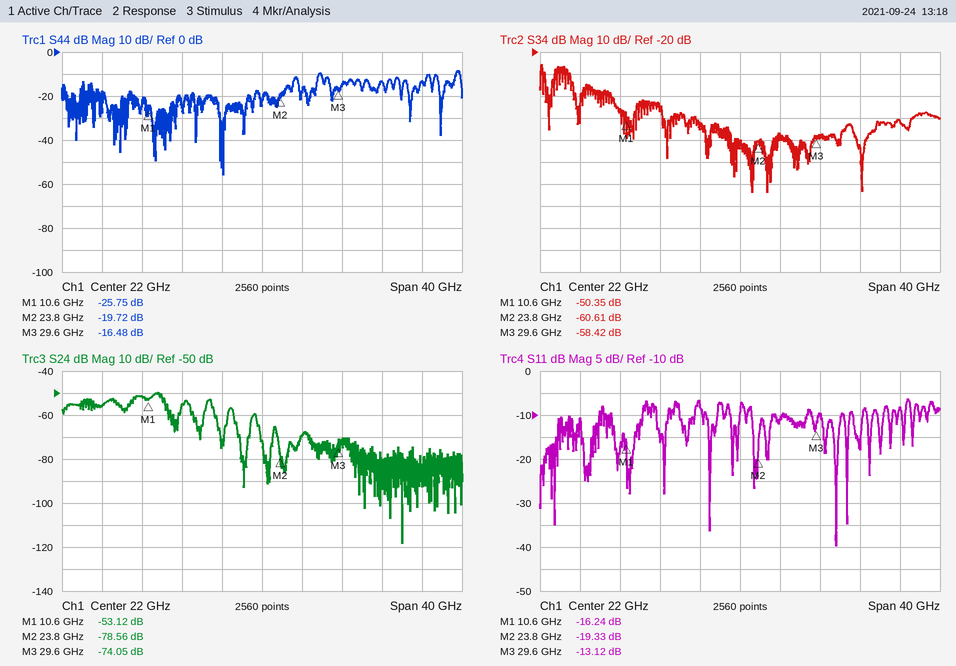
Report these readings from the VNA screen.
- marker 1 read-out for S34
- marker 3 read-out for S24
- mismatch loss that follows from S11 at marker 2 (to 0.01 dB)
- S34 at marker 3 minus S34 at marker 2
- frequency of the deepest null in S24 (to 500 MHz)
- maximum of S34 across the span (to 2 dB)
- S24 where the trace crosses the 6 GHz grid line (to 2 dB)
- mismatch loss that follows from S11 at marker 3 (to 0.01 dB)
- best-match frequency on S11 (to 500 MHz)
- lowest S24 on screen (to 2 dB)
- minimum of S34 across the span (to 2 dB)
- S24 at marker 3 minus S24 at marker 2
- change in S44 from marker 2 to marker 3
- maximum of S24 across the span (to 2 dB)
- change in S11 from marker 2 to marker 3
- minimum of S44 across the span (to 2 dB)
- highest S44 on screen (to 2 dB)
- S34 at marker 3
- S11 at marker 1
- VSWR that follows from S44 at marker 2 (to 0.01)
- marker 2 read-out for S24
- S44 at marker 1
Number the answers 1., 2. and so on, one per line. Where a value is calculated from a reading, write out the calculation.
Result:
1. -50.35 dB
2. -74.05 dB
3. −10 log10(1 − 10^(-19.33/10)) ≈ 0.05 dB
4. -58.42 − (-60.61) = 2.19 dB
5. 36.0 GHz
6. -26 dB
7. -56 dB
8. −10 log10(1 − 10^(-13.12/10)) ≈ 0.22 dB
9. 31.5 GHz
10. -118 dB
11. -84 dB
12. -74.05 − (-78.56) = 4.51 dB
13. -16.48 − (-19.72) = 3.24 dB
14. -50 dB
15. -13.12 − (-19.33) = 6.21 dB
16. -56 dB
17. -8 dB
18. -58.42 dB
19. -16.24 dB
20. (1 + 0.1033)/(1 − 0.1033) ≈ 1.23
21. -78.56 dB
22. -25.75 dB
